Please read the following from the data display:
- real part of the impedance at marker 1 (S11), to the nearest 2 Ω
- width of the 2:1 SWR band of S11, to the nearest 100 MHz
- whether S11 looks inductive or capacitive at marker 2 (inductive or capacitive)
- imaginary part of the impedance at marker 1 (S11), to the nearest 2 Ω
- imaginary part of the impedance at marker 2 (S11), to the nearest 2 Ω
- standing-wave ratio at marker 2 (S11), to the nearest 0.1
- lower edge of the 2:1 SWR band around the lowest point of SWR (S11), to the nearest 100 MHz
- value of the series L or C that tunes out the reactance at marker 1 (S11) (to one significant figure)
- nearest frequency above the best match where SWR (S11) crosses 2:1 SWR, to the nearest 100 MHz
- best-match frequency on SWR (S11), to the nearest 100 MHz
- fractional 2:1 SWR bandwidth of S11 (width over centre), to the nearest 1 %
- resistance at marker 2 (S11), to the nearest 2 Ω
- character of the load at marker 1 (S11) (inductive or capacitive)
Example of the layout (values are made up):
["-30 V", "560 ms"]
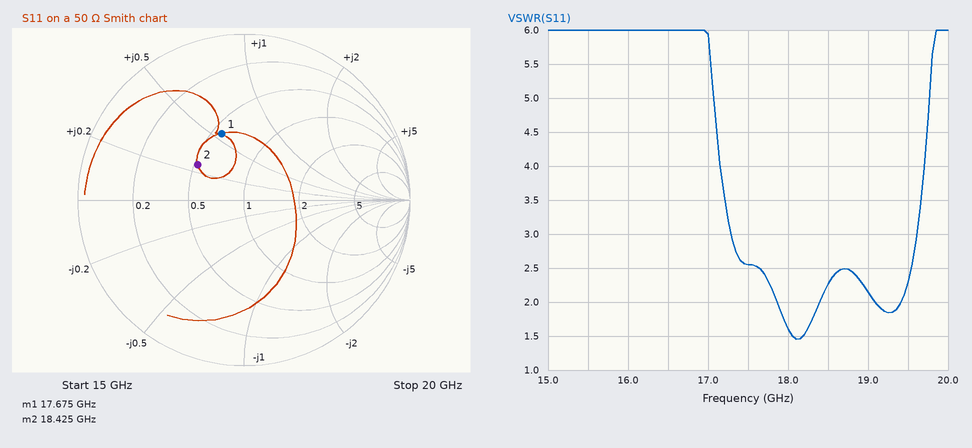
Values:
["28 Ω", "500 MHz", "inductive", "+28 Ω", "+12 Ω", "2.1", "17.9 GHz", "300 fF", "18.4 GHz", "18.1 GHz", "3 %", "26 Ω", "inductive"]
